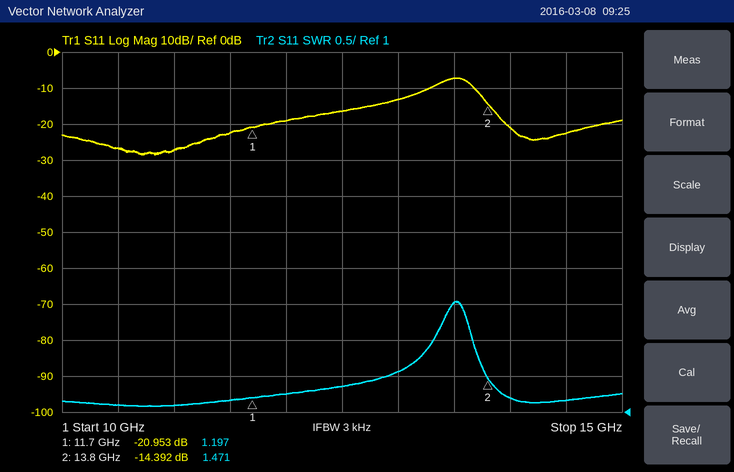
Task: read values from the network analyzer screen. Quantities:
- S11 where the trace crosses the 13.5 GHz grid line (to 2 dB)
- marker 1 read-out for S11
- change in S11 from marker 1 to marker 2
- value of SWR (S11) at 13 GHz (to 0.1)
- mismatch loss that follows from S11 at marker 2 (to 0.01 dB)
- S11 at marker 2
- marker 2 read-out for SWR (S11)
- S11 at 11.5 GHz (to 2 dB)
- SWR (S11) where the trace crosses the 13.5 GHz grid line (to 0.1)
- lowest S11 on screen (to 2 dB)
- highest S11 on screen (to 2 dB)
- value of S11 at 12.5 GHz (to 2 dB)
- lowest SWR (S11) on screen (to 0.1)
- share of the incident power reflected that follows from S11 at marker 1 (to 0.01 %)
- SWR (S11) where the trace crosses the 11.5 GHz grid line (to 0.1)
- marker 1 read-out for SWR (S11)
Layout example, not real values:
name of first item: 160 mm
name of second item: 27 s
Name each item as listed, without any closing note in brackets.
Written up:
S11 where the trace crosses the 13.5 GHz grid line: -8 dB
marker 1 read-out for S11: -20.953 dB
change in S11 from marker 1 to marker 2: 6.561 dB
value of SWR (S11) at 13 GHz: 1.6
mismatch loss that follows from S11 at marker 2: 0.16 dB
S11 at marker 2: -14.392 dB
marker 2 read-out for SWR: 1.471
S11 at 11.5 GHz: -22 dB
SWR (S11) where the trace crosses the 13.5 GHz grid line: 2.5
lowest S11 on screen: -28 dB
highest S11 on screen: -8 dB
value of S11 at 12.5 GHz: -16 dB
lowest SWR (S11) on screen: 1.1
share of the incident power reflected that follows from S11 at marker 1: 0.80 %
SWR (S11) where the trace crosses the 11.5 GHz grid line: 1.2
marker 1 read-out for SWR: 1.197
